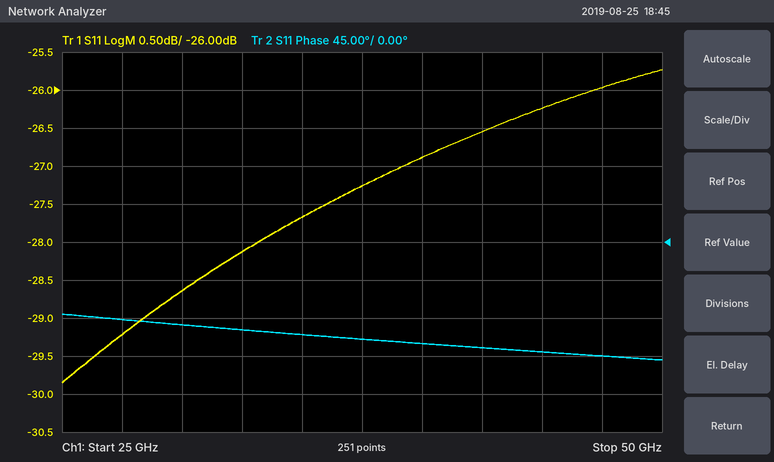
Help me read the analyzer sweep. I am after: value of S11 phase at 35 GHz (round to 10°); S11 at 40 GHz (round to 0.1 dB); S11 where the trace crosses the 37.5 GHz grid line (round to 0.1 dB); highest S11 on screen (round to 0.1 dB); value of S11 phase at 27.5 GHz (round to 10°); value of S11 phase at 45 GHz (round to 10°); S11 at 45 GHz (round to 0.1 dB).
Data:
-110°
-26.9 dB
-27.3 dB
-25.7 dB
-90°
-130°
-26.2 dB
